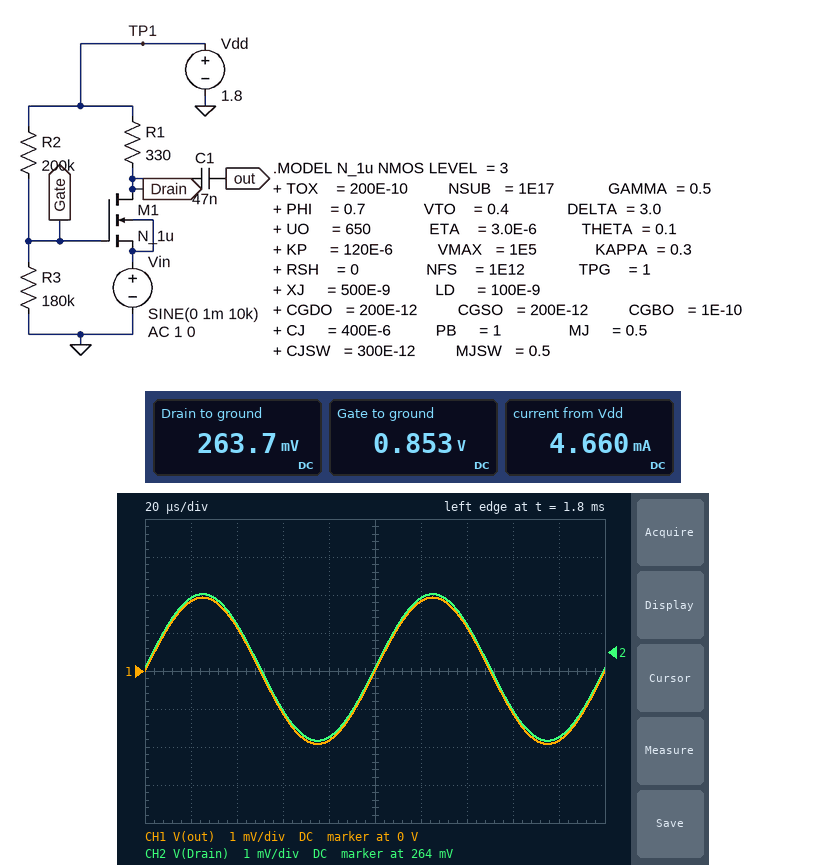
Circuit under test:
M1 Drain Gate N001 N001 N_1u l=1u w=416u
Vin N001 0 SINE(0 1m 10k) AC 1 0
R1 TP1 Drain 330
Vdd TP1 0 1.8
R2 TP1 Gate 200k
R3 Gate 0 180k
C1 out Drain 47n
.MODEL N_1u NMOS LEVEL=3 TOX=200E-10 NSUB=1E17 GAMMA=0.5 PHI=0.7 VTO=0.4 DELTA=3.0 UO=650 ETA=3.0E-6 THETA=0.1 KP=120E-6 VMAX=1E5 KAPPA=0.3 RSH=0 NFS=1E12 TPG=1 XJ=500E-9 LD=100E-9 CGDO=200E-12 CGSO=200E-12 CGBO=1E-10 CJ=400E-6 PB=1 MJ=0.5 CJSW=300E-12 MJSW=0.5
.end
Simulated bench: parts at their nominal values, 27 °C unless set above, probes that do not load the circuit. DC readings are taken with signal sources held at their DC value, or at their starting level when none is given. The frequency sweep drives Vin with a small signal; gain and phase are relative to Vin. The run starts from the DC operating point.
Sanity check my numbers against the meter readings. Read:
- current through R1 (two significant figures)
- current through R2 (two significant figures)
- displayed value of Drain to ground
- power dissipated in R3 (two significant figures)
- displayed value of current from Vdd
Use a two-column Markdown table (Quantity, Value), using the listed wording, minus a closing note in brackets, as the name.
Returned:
| Quantity | Value |
|---|---|
| current through R1 | 4.7 mA |
| current through R2 | 4.7 µA |
| displayed value of Drain to ground | 263.7 mV |
| power dissipated in R3 | 4.0 µW |
| displayed value of current from Vdd | 4.660 mA |
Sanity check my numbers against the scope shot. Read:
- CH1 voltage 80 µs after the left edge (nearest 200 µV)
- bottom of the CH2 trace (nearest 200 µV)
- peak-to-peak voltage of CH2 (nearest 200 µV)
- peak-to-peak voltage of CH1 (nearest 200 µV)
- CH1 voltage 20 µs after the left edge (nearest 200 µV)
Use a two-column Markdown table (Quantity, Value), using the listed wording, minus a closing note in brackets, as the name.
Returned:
| Quantity | Value |
|---|---|
| CH1 voltage 80 µs after the left edge | -1.8 mV |
| bottom of the CH2 trace | 261.6 mV |
| peak-to-peak voltage of CH2 | 3.8 mV |
| peak-to-peak voltage of CH1 | 3.8 mV |
| CH1 voltage 20 µs after the left edge | 1.8 mV |
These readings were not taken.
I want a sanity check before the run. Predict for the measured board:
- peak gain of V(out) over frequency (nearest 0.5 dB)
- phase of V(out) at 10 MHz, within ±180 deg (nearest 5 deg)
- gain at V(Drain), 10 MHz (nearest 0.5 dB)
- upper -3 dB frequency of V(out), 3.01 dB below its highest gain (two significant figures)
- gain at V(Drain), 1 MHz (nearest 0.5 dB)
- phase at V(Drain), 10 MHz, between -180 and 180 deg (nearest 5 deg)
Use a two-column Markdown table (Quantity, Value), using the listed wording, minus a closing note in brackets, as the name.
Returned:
| Quantity | Value |
|---|---|
| peak gain of V(out) over frequency | 5.5 dB |
| phase of V(out) at 10 MHz, within ±180 deg | -15 deg |
| gain at V(Drain), 10 MHz | -1.5 dB |
| upper -3 dB frequency of V(out), 3.01 dB below its highest gain | 2.1 MHz |
| gain at V(Drain), 1 MHz | 4.5 dB |
| phase at V(Drain), 10 MHz, between -180 and 180 deg | -15 deg |
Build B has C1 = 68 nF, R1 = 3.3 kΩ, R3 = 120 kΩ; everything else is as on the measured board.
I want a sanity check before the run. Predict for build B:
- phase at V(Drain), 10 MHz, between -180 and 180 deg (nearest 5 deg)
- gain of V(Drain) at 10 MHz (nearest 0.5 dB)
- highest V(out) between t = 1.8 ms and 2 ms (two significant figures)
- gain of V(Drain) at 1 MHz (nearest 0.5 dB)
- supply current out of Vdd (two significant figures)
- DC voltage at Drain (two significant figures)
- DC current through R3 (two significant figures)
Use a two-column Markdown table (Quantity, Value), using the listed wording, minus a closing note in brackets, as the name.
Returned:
| Quantity | Value |
|---|---|
| phase at V(Drain), 10 MHz, between -180 and 180 deg | 0 deg |
| gain of V(Drain) at 10 MHz | 0 dB |
| highest V(out) between t = 1.8 ms and 2 ms | 1.1 mV |
| gain of V(Drain) at 1 MHz | 0.5 dB |
| supply current out of Vdd | 540 µA |
| DC voltage at Drain | 29 mV |
| DC current through R3 | 5.6 µA |
